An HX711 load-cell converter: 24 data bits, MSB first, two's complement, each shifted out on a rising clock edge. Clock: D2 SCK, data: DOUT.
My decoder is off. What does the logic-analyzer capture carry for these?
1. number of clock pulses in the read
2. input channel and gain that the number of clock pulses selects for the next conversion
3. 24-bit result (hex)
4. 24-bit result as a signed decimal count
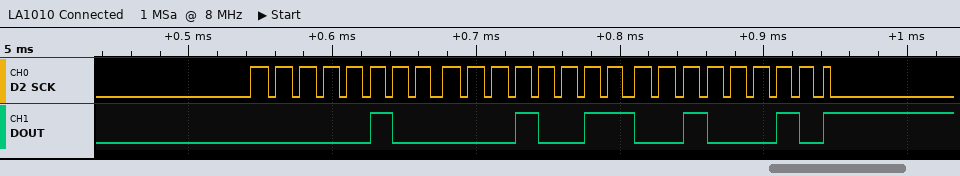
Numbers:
25
channel A, gain 128
0x041322
267042
